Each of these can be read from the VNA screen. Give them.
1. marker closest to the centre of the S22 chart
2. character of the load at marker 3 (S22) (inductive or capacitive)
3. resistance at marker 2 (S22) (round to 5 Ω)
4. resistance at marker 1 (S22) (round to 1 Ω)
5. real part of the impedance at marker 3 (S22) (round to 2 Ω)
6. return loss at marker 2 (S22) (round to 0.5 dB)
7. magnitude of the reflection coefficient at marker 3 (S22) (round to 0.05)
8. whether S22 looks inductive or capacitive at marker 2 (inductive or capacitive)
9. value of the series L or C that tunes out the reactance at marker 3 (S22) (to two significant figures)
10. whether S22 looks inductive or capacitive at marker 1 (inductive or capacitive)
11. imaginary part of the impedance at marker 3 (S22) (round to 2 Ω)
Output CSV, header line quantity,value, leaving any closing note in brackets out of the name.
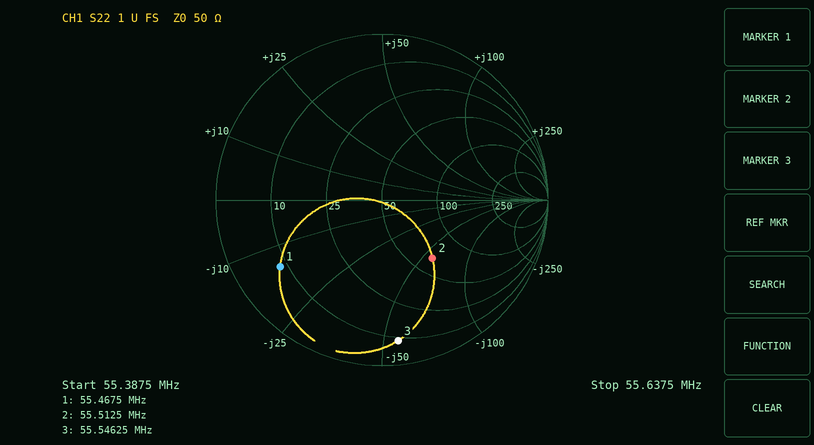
quantity,value
marker closest to the centre of the S22 chart,marker 2
character of the load at marker 3 (S22),capacitive
resistance at marker 2 (S22),65 Ω
resistance at marker 1 (S22),8 Ω
real part of the impedance at marker 3 (S22),8 Ω
return loss at marker 2 (S22),6.5 dB
magnitude of the reflection coefficient at marker 3 (S22),0.85
whether S22 looks inductive or capacitive at marker 2,capacitive
value of the series L or C that tunes out the reactance at marker 3 (S22),160 nH
whether S22 looks inductive or capacitive at marker 1,capacitive
imaginary part of the impedance at marker 3 (S22),-56 Ω
